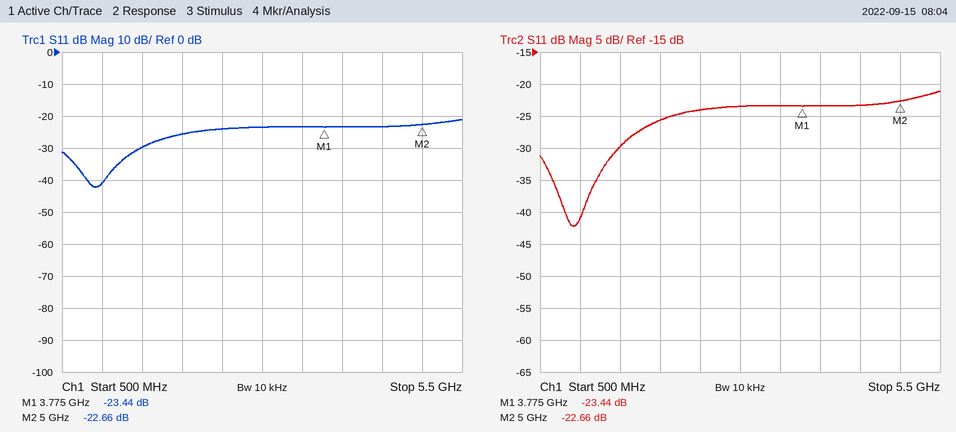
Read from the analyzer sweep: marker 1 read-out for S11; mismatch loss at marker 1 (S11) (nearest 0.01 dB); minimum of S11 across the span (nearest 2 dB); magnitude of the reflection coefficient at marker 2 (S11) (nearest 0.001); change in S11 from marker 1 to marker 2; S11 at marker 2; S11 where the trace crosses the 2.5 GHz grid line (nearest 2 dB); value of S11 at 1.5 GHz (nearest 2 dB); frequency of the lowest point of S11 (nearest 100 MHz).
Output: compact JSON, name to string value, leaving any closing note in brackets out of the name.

{"marker 1 read-out for S11": "-23.44 dB", "mismatch loss at marker 1 (S11)": "0.02 dB", "minimum of S11 across the span": "-42 dB", "magnitude of the reflection coefficient at marker 2 (S11)": "0.074", "change in S11 from marker 1 to marker 2": "0.78 dB", "S11 at marker 2": "-22.66 dB", "S11 where the trace crosses the 2.5 GHz grid line": "-24 dB", "value of S11 at 1.5 GHz": "-30 dB", "frequency of the lowest point of S11": "900 MHz"}
